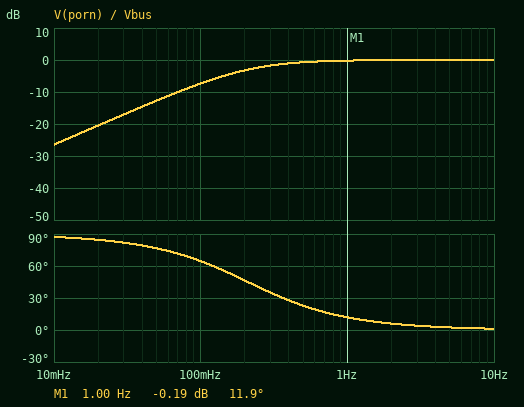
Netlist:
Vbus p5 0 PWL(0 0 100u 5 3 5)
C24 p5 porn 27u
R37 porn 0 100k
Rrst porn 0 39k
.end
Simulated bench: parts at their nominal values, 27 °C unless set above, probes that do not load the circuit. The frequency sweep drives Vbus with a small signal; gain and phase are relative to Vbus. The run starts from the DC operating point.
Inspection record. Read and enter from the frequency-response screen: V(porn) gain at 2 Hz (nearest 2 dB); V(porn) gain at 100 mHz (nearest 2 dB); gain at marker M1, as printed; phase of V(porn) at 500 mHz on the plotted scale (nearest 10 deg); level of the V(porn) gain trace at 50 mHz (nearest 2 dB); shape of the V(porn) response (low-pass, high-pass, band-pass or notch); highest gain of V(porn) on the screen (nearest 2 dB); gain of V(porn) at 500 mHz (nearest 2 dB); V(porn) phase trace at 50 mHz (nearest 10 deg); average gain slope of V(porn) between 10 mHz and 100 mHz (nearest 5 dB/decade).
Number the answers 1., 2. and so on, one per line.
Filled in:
1. 0 dB
2. -8 dB
3. -0.19 dB
4. 20 deg
5. -12 dB
6. high-pass
7. 0 dB
8. 0 dB
9. 80 deg
10. 20 dB/decade
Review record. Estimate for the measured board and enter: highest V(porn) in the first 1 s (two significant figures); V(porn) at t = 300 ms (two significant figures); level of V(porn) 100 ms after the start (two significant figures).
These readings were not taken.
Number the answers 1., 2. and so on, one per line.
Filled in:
1. 5.0 V
2. 3.4 V
3. 4.4 V
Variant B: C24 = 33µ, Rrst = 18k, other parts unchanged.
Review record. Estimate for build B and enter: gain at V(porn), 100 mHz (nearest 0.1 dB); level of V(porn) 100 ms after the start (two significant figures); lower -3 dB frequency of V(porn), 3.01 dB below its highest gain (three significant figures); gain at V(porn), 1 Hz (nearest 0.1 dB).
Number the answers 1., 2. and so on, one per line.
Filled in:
1. -10.4 dB
2. 4.1 V
3. 316 mHz
4. -0.4 dB
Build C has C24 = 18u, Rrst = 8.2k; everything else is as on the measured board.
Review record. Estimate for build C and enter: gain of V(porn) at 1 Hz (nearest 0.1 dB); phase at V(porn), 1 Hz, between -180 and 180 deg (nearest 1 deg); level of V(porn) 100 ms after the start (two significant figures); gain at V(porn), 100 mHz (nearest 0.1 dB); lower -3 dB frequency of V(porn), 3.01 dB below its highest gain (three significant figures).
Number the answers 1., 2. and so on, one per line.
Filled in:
1. -3.7 dB
2. 49 deg
3. 2.4 V
4. -21.4 dB
5. 1.17 Hz
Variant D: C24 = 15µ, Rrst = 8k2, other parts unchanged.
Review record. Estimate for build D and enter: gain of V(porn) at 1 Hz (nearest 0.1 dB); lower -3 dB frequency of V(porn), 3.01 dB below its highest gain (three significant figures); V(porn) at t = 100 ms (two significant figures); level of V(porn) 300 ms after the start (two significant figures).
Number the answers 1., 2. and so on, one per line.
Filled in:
1. -4.7 dB
2. 1.40 Hz
3. 2.1 V
4. 360 mV
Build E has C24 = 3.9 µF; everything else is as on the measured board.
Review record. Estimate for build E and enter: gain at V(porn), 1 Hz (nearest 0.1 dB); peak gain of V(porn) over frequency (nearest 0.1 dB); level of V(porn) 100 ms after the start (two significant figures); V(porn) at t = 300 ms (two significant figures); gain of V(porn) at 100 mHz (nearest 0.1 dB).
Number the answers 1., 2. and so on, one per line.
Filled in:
1. -4.9 dB
2. 0 dB
3. 2.0 V
4. 320 mV
5. -23.3 dB
